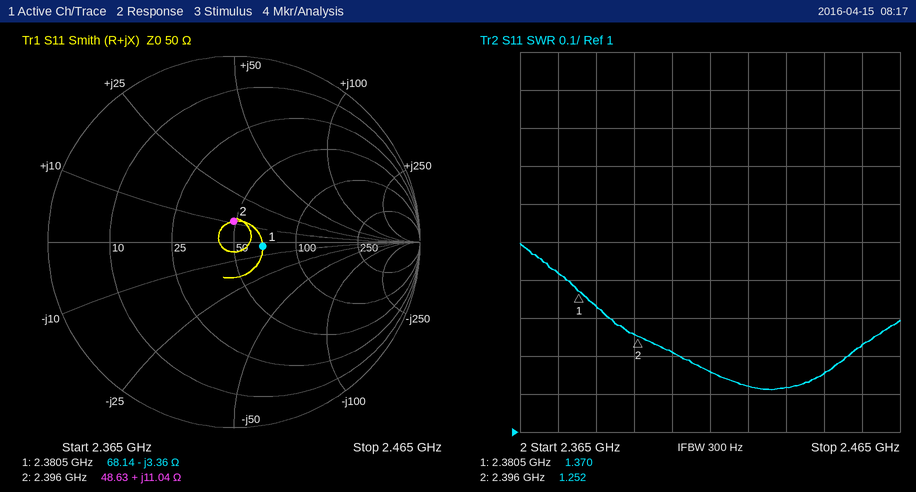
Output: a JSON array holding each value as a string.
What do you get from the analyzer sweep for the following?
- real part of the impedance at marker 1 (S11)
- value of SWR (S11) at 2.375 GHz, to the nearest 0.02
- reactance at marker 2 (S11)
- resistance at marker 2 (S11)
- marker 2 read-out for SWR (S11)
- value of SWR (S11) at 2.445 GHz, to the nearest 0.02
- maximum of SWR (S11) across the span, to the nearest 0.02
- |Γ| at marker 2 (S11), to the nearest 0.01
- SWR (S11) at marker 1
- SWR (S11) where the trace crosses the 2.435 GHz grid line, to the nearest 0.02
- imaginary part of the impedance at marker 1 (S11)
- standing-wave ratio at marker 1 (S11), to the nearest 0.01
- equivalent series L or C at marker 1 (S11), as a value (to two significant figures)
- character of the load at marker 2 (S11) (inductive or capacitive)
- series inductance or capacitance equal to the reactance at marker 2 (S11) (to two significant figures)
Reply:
["68.14 Ω", "1.42", "+11.04 Ω", "48.63 Ω", "1.252", "1.16", "1.50", "0.11", "1.370", "1.12", "-3.36 Ω", "1.37", "20 pF", "inductive", "730 pH"]
